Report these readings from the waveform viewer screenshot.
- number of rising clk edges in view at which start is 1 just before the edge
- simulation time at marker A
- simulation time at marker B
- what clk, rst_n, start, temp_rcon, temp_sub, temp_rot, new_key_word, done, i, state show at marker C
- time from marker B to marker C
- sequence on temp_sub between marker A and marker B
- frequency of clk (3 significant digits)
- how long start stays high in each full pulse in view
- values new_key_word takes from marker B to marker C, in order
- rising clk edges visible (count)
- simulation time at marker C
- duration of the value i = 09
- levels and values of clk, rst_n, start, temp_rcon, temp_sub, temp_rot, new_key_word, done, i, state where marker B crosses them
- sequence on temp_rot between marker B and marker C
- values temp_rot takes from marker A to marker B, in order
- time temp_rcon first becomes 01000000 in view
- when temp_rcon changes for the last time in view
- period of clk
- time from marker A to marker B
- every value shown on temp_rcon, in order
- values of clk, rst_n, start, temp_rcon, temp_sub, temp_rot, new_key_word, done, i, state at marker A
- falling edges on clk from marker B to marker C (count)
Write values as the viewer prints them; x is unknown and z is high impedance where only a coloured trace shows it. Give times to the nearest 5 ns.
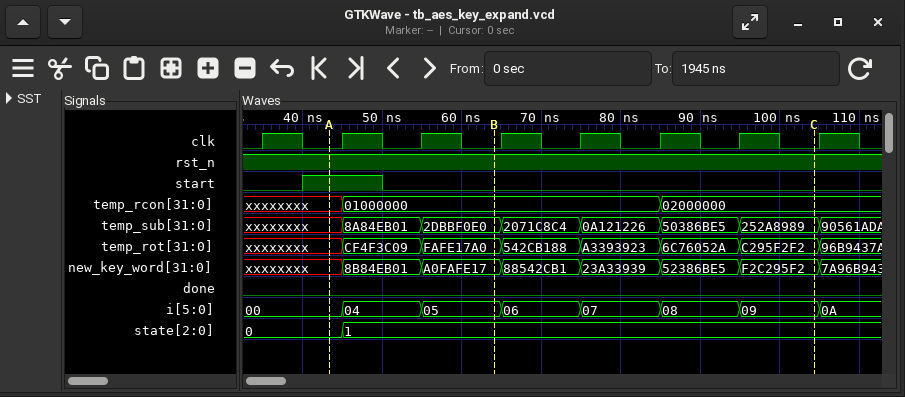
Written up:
1
45 ns
65 ns
clk=0, rst_n=1, start=0, temp_rcon=02000000, temp_sub=252A8989, temp_rot=C295F2F2, new_key_word=F2C295F2, done=0, i=09, state=1
40 ns
xxxxxxxx, 8A84EB01, 2DBBF0E0
100 MHz
10 ns
A0FAFE17, 88542CB1, 23A33939, 52386BE5, F2C295F2
8
105 ns
10 ns
clk=0, rst_n=1, start=0, temp_rcon=01000000, temp_sub=2DBBF0E0, temp_rot=FAFE17A0, new_key_word=A0FAFE17, done=0, i=05, state=1
FAFE17A0, 542CB188, A3393923, 6C76052A, C295F2F2
xxxxxxxx, CF4F3C09, FAFE17A0
45 ns
85 ns
10 ns
20 ns
xxxxxxxx, 01000000, 02000000
clk=0, rst_n=1, start=1, temp_rcon=xxxxxxxx, temp_sub=xxxxxxxx, temp_rot=xxxxxxxx, new_key_word=xxxxxxxx, done=0, i=00, state=0
4
